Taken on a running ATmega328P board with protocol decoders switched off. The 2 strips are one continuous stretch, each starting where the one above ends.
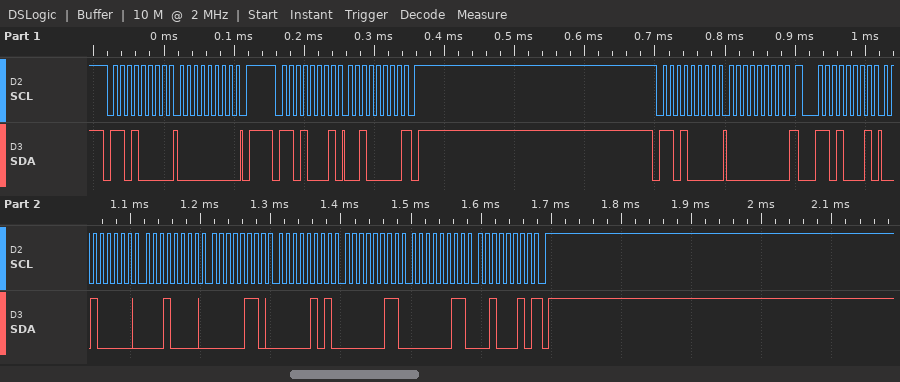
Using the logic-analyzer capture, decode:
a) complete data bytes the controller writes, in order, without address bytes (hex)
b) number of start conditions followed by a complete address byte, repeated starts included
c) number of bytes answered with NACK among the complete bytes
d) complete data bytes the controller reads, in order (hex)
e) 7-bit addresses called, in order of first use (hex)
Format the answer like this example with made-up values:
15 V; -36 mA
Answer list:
00 00; 4; 2; 20 20 10 06 05 03 03 22; 0x68
